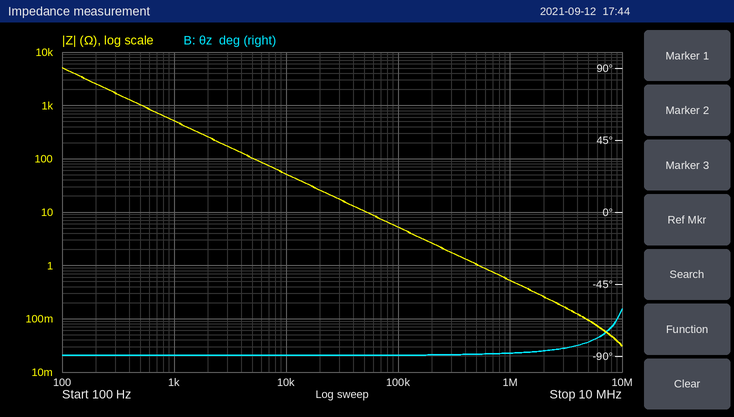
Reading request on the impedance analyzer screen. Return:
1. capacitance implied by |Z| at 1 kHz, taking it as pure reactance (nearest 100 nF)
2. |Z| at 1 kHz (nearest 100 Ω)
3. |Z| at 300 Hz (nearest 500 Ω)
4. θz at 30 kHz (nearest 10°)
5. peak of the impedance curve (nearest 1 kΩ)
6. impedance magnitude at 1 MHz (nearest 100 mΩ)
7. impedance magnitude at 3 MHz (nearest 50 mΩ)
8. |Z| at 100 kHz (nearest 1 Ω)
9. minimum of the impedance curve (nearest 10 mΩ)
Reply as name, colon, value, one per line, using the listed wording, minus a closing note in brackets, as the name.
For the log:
capacitance implied by |Z| at 1 kHz, taking it as pure reactance: 300 nF
|Z| at 1 kHz: 500 Ω
|Z| at 300 Hz: 1.5 kΩ
θz at 30 kHz: -90°
peak of the impedance curve: 5 kΩ
impedance magnitude at 1 MHz: 500 mΩ
impedance magnitude at 3 MHz: 150 mΩ
|Z| at 100 kHz: 5 Ω
minimum of the impedance curve: 30 mΩ
